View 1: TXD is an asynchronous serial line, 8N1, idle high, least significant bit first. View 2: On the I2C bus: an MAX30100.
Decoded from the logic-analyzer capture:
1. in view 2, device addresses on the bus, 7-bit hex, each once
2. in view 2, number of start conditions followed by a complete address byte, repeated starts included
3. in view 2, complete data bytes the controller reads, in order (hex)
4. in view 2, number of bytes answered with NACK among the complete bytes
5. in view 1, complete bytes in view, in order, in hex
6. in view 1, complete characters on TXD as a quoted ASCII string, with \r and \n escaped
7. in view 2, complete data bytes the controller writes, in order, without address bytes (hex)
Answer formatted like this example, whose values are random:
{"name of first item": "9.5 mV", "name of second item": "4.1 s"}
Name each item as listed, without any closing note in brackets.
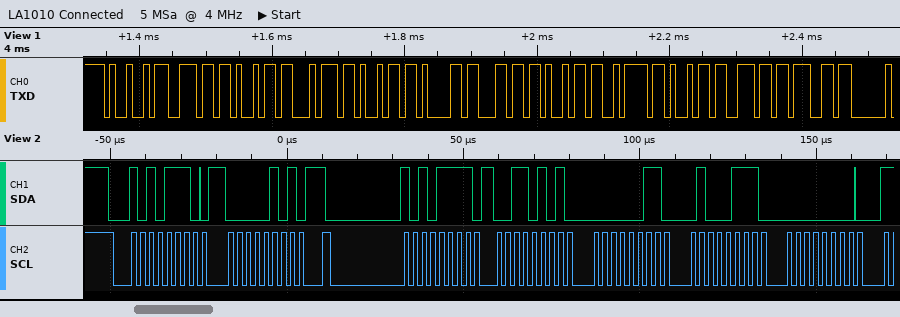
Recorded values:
{"in view 2, device addresses on the bus, 7-bit hex, each once": "0x57", "in view 2, number of start conditions followed by a complete address byte, repeated starts included": "2", "in view 2, complete data bytes the controller reads, in order": "35 03 47 00", "in view 2, number of bytes answered with NACK among the complete bytes": "0", "in view 1, complete bytes in view, in order, in hex": "49 6E 69 74 69 61 6C 69 7A 69 6E 67", "in view 1, complete characters on TXD as a quoted ASCII string, with \\r and \\n escaped": "\"Initializing\"", "in view 2, complete data bytes the controller writes, in order, without address bytes": "05"}
